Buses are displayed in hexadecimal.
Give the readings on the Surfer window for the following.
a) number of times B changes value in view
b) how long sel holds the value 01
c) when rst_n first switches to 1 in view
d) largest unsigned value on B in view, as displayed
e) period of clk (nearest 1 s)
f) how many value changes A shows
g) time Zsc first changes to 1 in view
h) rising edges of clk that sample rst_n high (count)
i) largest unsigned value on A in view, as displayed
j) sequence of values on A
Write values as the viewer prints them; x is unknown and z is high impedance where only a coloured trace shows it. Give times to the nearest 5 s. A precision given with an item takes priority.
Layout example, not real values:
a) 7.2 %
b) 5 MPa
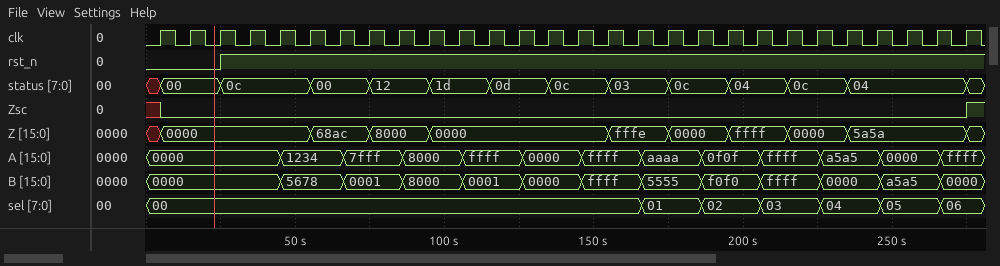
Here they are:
a) 12
b) 20 s
c) 25 s
d) ffff
e) 10 s
f) 12
g) 275 s
h) 25
i) ffff
j) 0000, 1234, 7fff, 8000, ffff, 0000, ffff, aaaa, 0f0f, ffff, a5a5, 0000, ffff
